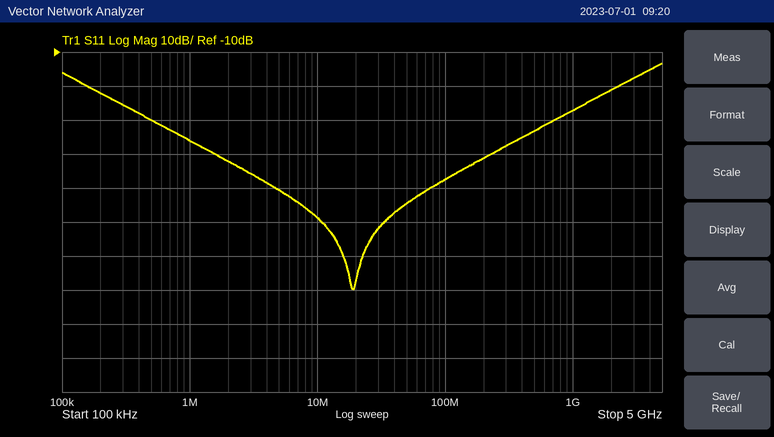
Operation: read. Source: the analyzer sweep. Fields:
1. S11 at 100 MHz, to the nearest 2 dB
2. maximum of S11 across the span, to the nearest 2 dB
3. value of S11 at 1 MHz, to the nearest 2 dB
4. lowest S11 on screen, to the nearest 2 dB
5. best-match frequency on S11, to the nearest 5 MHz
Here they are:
-48 dB
-14 dB
-36 dB
-80 dB
20 MHz
